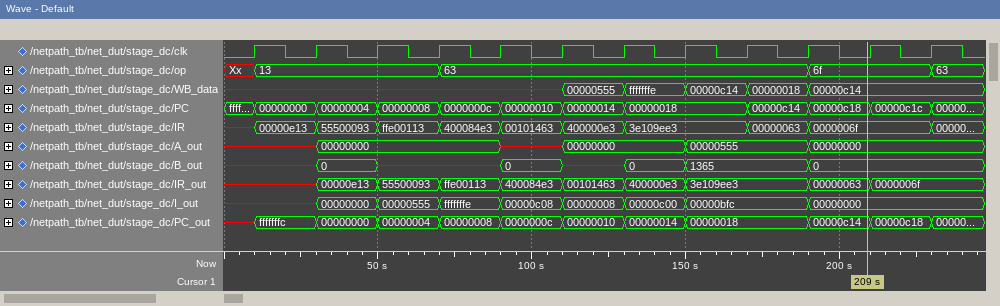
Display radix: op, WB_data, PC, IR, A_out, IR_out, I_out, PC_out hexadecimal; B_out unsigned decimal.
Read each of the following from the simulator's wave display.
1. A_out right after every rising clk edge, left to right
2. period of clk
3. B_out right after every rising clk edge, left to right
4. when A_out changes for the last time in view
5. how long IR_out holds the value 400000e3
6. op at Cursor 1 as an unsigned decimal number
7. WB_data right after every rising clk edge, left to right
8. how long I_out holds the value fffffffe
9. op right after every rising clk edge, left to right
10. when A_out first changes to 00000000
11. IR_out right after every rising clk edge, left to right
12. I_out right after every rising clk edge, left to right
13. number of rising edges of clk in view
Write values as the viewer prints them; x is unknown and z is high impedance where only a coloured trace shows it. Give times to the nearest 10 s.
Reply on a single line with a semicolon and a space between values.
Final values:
x, 00000000, 00000000, 00000000, x, 00000000, 00000000, 00000555, 00000555, 00000000, 00000000, 00000000; 20 s; x, 0, x, x, 0, x, 0, 1365, 1365, 0, 0, 0; 190 s; 20 s; 111; x, x, x, x, x, 00000555, fffffffe, 00000c14, 00000018, 00000c14, 00000c14, 00000c14; 20 s; 13, 13, 13, 63, 63, 63, 63, 63, 63, 6f, 6f, 63; 30 s; x, 00000e13, 55500093, ffe00113, 400084e3, 00101463, 400000e3, 3e109ee3, 3e109ee3, 00000063, 0000006f, 0000006f; x, 00000000, 00000555, fffffffe, 00000c08, 00000008, 00000c00, 00000bfc, 00000bfc, 00000000, 00000000, 00000000; 12
